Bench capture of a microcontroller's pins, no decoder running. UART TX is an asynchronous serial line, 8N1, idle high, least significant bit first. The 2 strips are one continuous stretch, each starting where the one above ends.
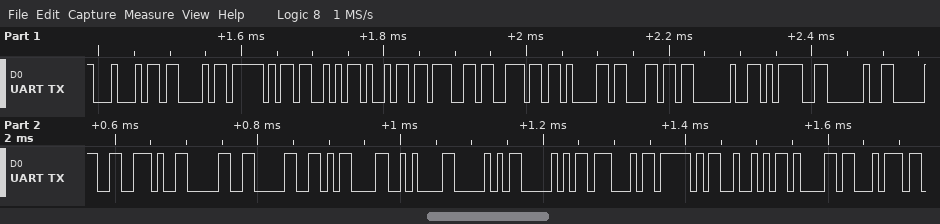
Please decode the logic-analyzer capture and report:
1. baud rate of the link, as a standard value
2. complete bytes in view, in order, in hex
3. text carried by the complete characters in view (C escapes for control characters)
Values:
115200 baud
0x44 0x43 0x5F 0x53 0x69 0x67 0x6E 0x61 0x6C 0x20 0x3D 0x20 0x30 0x2E 0x30 0x30 0x0D 0x0A 0x50 0x50 0x47 0x5F 0x52 0x61 0x74
"DC_Signal = 0.00\r\nPPG_Rat"
